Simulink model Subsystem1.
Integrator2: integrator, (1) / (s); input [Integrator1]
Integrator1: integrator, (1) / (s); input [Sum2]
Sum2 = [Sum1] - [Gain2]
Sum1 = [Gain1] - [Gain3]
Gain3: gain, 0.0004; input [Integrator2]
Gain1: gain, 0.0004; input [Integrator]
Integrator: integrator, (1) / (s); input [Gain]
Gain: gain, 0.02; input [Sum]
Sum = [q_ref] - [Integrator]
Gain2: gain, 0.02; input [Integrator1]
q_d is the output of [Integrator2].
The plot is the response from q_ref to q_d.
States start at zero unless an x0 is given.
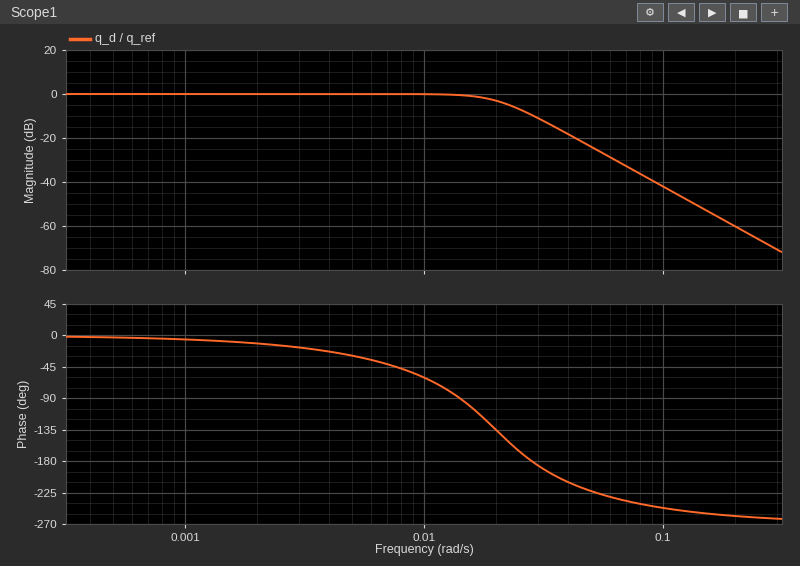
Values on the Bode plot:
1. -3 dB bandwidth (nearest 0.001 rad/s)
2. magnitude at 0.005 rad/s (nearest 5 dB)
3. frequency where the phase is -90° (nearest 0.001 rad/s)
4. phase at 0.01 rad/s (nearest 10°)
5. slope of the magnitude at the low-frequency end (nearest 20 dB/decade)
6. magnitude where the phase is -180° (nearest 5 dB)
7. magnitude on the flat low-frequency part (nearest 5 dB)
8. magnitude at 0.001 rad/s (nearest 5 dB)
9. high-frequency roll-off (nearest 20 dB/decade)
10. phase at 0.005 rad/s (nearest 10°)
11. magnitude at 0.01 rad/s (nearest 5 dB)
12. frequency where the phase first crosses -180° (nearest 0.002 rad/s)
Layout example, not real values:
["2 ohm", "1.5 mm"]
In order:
["0.020 rad/s", "0 dB", "0.014 rad/s", "-60°", "0 dB/decade", "-10 dB", "0 dB", "0 dB", "-60 dB/decade", "-30°", "0 dB", "0.028 rad/s"]
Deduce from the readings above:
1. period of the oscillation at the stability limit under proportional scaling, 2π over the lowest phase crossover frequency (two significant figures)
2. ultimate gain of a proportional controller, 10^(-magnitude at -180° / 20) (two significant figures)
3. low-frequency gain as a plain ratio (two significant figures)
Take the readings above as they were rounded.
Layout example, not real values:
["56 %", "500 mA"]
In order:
["220 s", "3.2", "1.0"]
